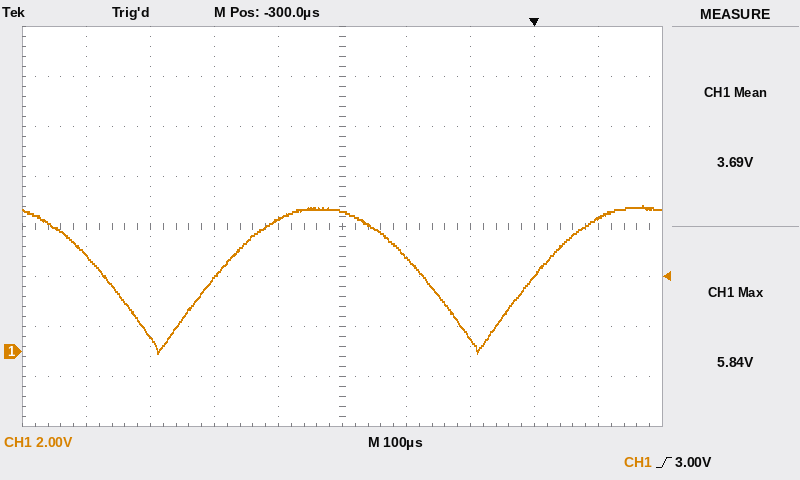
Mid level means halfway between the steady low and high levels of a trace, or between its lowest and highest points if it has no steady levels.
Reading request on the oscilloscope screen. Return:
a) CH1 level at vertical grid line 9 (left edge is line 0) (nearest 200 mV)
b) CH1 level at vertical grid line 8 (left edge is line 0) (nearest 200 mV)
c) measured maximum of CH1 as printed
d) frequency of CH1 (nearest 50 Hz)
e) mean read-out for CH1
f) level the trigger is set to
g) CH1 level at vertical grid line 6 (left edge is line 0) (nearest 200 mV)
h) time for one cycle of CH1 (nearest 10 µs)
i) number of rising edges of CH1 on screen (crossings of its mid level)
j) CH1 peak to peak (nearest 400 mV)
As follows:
5.4 V
3.0 V
5.84 V
2.00 kHz
3.69 V
3.00 V
3.8 V
500 µs
2
6.0 V
